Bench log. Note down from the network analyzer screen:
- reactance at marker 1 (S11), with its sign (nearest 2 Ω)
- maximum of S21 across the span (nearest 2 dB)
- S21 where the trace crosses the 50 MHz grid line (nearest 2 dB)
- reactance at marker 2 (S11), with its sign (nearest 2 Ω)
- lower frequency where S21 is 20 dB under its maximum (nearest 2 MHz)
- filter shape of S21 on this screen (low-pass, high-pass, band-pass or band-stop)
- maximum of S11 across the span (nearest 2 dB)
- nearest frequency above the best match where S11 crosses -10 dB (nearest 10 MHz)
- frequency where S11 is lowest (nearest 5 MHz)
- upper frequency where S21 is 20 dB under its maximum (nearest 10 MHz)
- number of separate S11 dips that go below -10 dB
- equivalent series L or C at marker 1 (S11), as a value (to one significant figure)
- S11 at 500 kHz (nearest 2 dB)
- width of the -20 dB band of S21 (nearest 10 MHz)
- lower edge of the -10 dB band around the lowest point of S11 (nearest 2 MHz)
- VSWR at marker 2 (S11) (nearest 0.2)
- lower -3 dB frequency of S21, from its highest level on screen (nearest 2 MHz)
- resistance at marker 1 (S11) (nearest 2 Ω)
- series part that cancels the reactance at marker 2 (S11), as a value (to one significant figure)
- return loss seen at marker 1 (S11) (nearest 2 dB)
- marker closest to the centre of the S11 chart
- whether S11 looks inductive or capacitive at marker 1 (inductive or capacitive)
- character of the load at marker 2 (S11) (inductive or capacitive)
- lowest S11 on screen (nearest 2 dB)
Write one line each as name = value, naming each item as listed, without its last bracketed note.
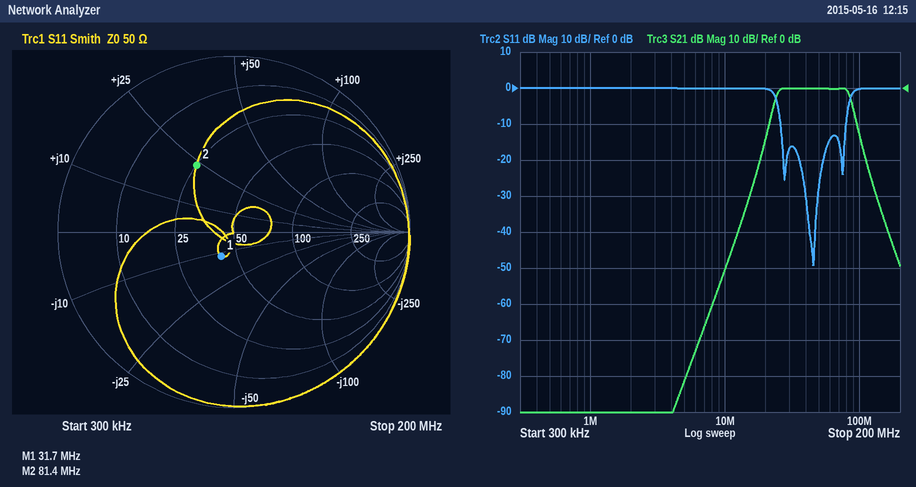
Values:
reactance at marker 1 (S11), with its sign = -12 Ω
maximum of S21 across the span = 0 dB
S21 where the trace crosses the 50 MHz grid line = 0 dB
reactance at marker 2 (S11), with its sign = +24 Ω
lower frequency where S21 is 20 dB under its maximum = 18 MHz
filter shape of S21 on this screen = band-pass
maximum of S11 across the span = 0 dB
nearest frequency above the best match where S11 crosses -10 dB = 80 MHz
frequency where S11 is lowest = 45 MHz
upper frequency where S21 is 20 dB under its maximum = 110 MHz
number of separate S11 dips that go below -10 dB = 3
equivalent series L or C at marker 1 (S11), as a value = 400 pF
S11 at 500 kHz = 0 dB
width of the -20 dB band of S21 = 90 MHz
lower edge of the -10 dB band around the lowest point of S11 = 26 MHz
VSWR at marker 2 (S11) = 2.6
lower -3 dB frequency of S21, from its highest level on screen = 24 MHz
resistance at marker 1 (S11) = 42 Ω
series part that cancels the reactance at marker 2 (S11), as a value = 80 pF
return loss seen at marker 1 (S11) = 16 dB
marker closest to the centre of the S11 chart = marker 1
whether S11 looks inductive or capacitive at marker 1 = capacitive
character of the load at marker 2 (S11) = inductive
lowest S11 on screen = -50 dB
